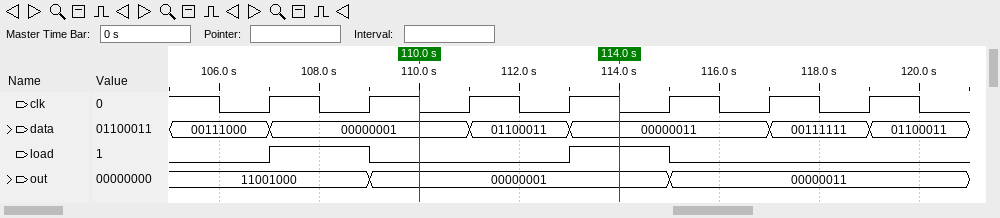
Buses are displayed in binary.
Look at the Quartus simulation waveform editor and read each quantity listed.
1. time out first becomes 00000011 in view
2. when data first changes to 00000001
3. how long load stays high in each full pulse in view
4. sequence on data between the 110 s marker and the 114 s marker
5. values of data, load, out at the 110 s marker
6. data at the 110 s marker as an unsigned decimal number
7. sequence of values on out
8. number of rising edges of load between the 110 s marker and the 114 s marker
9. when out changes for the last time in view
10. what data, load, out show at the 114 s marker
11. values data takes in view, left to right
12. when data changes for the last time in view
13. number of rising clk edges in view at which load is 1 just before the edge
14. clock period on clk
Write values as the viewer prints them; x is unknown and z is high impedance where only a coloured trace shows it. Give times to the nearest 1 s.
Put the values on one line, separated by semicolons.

115 s; 107 s; 2 s, 2 s; 00000001, 01100011, 00000011; data=00000001, load=0, out=00000001; 1; 11001000, 00000001, 00000011; 1; 115 s; data=00000011, load=1, out=00000001; 00111000, 00000001, 01100011, 00000011, 00111111, 01100011; 119 s; 2; 2 s
